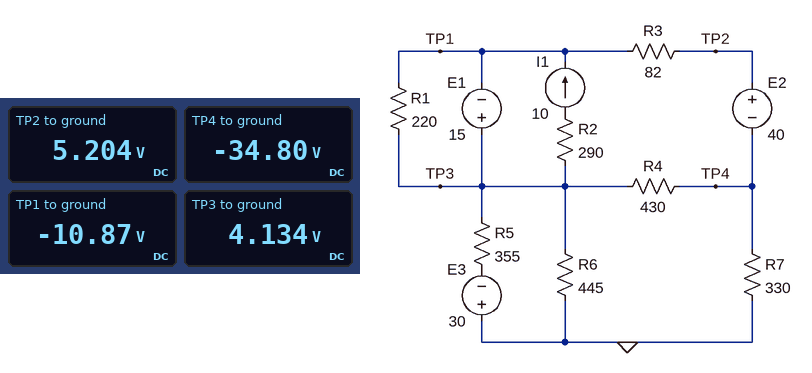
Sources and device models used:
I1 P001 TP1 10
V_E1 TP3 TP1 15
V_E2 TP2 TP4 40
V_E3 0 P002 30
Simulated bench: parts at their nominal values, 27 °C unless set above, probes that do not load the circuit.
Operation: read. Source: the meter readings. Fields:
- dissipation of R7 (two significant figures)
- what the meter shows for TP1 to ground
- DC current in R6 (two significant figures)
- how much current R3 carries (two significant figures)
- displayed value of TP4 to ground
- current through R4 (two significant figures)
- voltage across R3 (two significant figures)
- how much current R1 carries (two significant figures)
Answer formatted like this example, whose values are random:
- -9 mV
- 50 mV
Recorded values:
- 3.7 W
- -10.87 V
- 9.3 mA
- 200 mA
- -34.80 V
- 91 mA
- 16 V
- 68 mA
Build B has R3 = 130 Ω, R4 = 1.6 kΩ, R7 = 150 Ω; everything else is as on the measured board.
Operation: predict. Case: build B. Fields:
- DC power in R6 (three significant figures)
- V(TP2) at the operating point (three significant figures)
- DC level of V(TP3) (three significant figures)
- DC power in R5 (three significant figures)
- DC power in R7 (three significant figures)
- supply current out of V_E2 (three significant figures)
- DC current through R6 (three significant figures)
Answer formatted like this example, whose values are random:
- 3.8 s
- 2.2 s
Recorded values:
- 315 mW
- 18.3 V
- 11.8 V
- 4.93 W
- 3.13 W
- 165 mA
- 26.6 mA
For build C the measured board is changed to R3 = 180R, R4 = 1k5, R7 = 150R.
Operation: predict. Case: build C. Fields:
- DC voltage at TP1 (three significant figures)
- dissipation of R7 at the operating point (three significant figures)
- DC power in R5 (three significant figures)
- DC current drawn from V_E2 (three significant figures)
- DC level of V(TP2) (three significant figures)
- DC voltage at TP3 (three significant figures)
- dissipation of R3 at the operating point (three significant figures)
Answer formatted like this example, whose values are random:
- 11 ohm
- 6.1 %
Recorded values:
- -6.12 V
- 2.51 W
- 4.26 W
- 148 mA
- 20.6 V
- 8.88 V
- 3.96 W
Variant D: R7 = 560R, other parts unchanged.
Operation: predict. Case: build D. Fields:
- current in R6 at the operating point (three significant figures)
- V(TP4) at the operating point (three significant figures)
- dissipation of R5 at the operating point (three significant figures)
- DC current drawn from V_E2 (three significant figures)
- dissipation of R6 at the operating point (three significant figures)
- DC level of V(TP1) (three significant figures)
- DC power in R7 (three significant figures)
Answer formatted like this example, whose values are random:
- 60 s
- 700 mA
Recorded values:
- 3.73 mA
- -42.6 V
- 2.26 W
- 171 mA
- 6.20 mW
- -16.7 V
- 3.24 W
